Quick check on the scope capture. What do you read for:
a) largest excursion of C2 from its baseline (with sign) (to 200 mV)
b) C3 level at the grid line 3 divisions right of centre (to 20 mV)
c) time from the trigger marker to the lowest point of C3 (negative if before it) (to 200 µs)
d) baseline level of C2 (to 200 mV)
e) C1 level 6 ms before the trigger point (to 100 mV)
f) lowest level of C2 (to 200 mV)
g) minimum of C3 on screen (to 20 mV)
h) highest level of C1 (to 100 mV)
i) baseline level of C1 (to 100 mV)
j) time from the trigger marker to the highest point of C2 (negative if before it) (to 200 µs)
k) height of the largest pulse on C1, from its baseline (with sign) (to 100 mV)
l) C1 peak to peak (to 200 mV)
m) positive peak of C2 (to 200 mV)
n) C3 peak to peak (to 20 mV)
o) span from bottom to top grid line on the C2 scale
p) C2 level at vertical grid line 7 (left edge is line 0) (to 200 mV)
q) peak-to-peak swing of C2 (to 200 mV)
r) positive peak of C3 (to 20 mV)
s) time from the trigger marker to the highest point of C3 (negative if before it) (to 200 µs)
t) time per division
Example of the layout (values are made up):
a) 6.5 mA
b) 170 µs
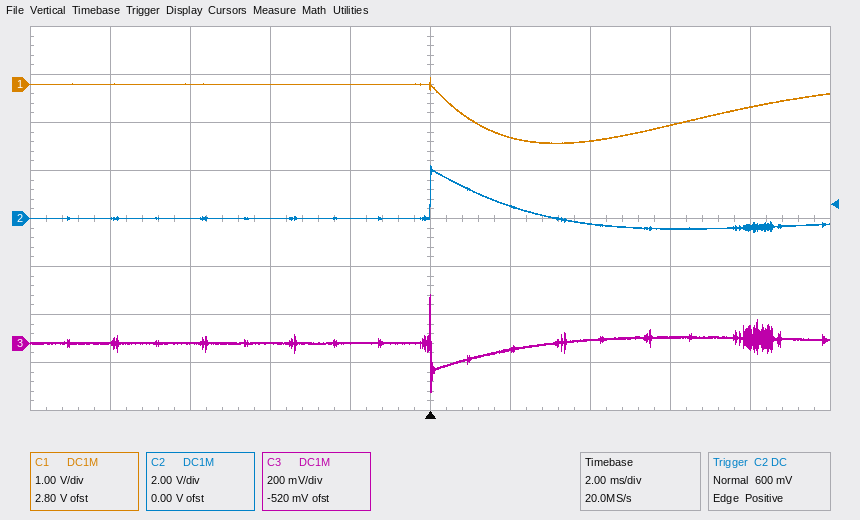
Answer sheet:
a) +2.2 V
b) 20 mV
c) 0.0 ms
d) 0.0 V
e) 0.0 V
f) -600 mV
g) -200 mV
h) 100 mV
i) 0.0 V
j) 0.0 ms
k) -1.2 V
l) 1.4 V
m) 2.2 V
n) 400 mV
o) 16 V
p) -200 mV
q) 2.8 V
r) 200 mV
s) 0.0 ms
t) 2 ms
